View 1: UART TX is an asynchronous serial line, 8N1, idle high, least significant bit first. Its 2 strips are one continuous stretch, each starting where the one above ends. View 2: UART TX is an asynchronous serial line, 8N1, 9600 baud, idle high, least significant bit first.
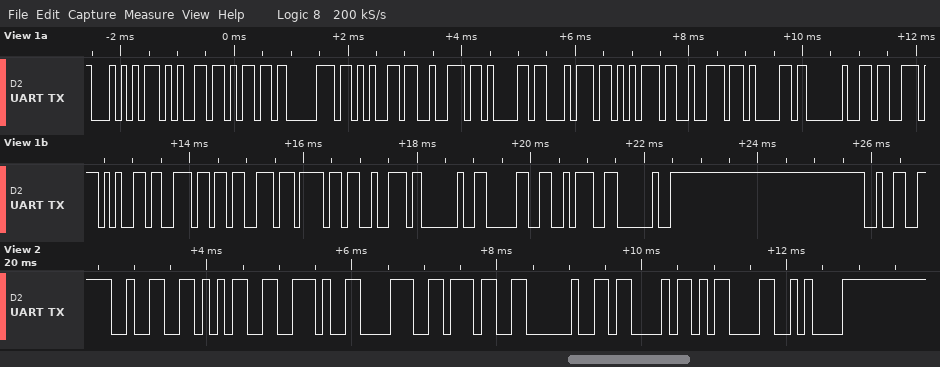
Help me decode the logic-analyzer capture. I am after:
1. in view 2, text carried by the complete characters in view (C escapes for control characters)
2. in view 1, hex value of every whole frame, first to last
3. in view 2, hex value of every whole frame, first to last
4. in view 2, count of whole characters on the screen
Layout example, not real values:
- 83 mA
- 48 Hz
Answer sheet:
- "25.87 C\r\n"
- 0x54 0x65 0x6D 0x70 0x65 0x72 0x61 0x74 0x75 0x72 0x61 0x20 0x73 0x65 0x6E 0x73 0x6F 0x72 0x20 0x30 0x3A 0x20 0x32
- 32 35 2E 38 37 20 43 0D 0A
- 9
